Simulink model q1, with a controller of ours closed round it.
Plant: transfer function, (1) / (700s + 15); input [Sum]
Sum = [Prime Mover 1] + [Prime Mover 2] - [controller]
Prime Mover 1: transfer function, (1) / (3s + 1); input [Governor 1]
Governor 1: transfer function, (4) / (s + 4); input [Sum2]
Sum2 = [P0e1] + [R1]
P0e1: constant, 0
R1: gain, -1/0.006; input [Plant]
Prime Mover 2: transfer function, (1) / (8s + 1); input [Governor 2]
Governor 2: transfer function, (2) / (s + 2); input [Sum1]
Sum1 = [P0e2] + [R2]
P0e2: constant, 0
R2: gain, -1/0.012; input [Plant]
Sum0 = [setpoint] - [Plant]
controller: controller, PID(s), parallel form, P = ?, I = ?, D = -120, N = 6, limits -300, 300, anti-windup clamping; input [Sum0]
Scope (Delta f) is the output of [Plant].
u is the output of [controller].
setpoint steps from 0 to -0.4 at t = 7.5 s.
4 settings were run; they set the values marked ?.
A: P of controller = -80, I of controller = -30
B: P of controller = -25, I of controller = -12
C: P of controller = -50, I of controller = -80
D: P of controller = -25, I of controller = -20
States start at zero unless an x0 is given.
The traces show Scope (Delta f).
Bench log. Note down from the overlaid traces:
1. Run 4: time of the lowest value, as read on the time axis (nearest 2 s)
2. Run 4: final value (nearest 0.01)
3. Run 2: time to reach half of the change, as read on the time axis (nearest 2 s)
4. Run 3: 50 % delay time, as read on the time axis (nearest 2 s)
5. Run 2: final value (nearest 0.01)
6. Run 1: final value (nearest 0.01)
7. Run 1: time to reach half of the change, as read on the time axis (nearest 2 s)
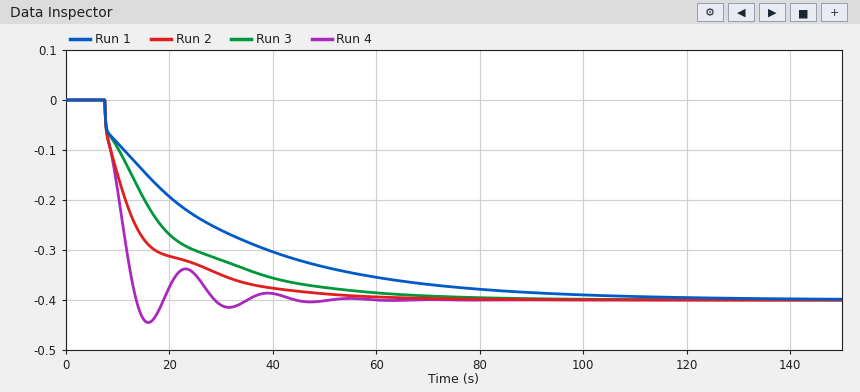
16 s
-0.40
12 s
16 s
-0.40
-0.40
20 s
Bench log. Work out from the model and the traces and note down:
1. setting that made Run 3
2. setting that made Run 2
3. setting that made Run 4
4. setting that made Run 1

D
A
C
B
